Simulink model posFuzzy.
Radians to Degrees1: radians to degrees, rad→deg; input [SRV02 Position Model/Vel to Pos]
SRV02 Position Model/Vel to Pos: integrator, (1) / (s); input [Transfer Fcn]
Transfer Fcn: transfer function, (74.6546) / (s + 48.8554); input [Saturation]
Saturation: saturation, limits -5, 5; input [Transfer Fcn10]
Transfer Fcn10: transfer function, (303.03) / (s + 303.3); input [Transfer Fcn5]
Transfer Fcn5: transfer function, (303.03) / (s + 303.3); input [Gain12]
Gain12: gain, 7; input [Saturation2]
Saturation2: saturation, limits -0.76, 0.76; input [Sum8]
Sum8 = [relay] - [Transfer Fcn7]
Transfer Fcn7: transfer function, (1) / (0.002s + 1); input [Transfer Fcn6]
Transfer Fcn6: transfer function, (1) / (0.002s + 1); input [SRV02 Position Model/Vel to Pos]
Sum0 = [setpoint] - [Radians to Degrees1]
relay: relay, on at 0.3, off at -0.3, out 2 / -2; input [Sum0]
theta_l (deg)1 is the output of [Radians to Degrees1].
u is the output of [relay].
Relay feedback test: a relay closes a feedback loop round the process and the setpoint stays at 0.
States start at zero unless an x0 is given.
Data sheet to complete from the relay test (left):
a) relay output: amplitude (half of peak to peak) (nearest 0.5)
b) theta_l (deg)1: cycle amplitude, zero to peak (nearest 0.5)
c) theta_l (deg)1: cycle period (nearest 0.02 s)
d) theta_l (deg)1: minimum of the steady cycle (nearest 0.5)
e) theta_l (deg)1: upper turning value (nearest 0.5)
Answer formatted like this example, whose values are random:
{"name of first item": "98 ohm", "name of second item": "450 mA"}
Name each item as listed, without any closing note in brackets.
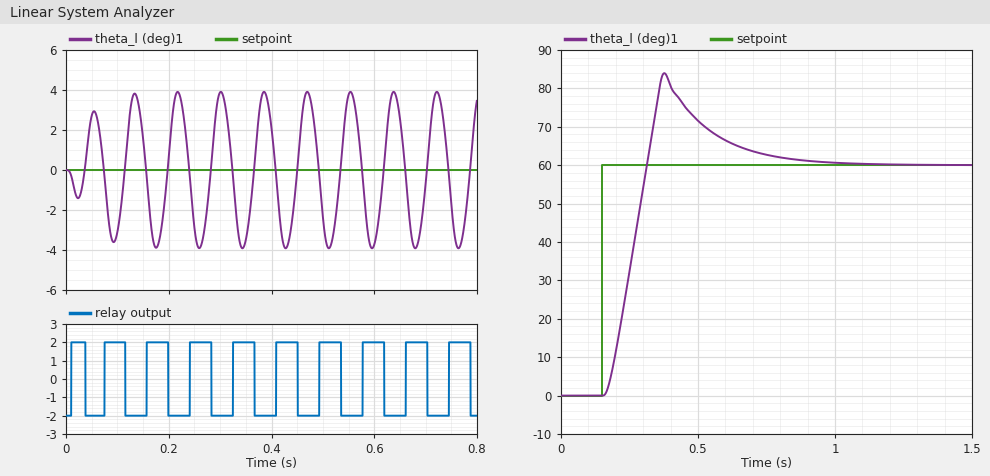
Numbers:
{"relay output: amplitude (half of peak to peak)": "2.0", "theta_l (deg)1: cycle amplitude, zero to peak": "4.0", "theta_l (deg)1: cycle period": "0.08 s", "theta_l (deg)1: minimum of the steady cycle": "-4.0", "theta_l (deg)1: upper turning value": "4.0"}
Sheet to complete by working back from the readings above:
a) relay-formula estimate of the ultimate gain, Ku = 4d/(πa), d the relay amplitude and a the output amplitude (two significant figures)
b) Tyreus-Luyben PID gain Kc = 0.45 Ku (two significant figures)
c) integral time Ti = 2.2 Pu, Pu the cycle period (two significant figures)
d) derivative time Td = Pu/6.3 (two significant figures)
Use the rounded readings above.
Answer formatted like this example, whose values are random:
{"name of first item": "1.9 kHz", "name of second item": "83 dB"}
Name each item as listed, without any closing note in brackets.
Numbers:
{"relay-formula estimate of the ultimate gain, Ku = 4d/(πa), d the relay amplitude and a the output amplitude": "0.64", "Tyreus-Luyben PID gain Kc = 0.45 Ku": "0.29", "integral time Ti = 2.2 Pu, Pu the cycle period": "0.18 s", "derivative time Td = Pu/6.3": "0.013 s"}
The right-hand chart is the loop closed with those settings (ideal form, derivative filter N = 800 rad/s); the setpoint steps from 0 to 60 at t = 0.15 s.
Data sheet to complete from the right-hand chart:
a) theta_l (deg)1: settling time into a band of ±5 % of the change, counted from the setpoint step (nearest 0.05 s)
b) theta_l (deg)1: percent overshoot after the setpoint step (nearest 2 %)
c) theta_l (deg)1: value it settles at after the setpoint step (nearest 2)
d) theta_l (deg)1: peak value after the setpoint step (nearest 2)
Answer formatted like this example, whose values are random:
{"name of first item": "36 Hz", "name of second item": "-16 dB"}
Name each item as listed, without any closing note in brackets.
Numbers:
{"theta_l (deg)1: settling time into a band of ±5 % of the change, counted from the setpoint step": "0.60 s", "theta_l (deg)1: percent overshoot after the setpoint step": "40 %", "theta_l (deg)1: value it settles at after the setpoint step": "60", "theta_l (deg)1: peak value after the setpoint step": "84"}
